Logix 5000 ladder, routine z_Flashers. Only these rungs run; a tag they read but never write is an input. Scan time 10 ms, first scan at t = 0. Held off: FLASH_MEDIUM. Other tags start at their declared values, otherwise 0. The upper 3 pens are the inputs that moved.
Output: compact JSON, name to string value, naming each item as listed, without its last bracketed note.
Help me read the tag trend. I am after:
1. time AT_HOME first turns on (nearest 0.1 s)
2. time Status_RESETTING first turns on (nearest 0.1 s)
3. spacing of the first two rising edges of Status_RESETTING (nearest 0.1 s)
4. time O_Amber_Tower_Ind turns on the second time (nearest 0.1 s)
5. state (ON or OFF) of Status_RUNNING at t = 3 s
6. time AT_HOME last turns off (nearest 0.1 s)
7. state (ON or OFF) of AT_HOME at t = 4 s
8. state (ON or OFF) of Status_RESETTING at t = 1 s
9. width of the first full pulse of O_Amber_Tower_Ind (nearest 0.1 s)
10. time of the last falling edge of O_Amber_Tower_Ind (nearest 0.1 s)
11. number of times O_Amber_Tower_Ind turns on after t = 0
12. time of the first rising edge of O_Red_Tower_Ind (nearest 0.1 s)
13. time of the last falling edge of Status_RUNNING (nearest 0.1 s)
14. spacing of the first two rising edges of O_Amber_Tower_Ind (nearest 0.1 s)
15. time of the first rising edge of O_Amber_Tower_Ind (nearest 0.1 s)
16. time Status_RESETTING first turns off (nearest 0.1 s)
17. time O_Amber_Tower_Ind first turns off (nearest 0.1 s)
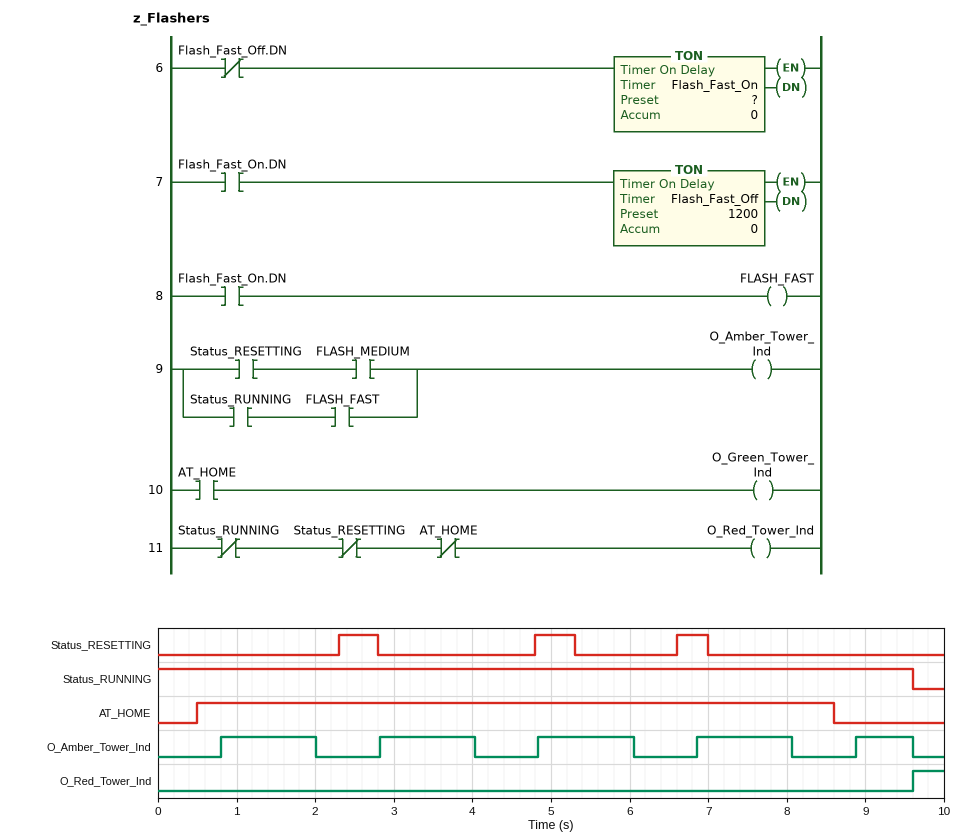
{"time AT_HOME first turns on": "0.5 s", "time Status_RESETTING first turns on": "2.3 s", "spacing of the first two rising edges of Status_RESETTING": "2.5 s", "time O_Amber_Tower_Ind turns on the second time": "2.8 s", "state (ON or OFF) of Status_RUNNING at t = 3 s": "ON", "time AT_HOME last turns off": "8.6 s", "state (ON or OFF) of AT_HOME at t = 4 s": "ON", "state (ON or OFF) of Status_RESETTING at t = 1 s": "OFF", "width of the first full pulse of O_Amber_Tower_Ind": "1.2 s", "time of the last falling edge of O_Amber_Tower_Ind": "9.6 s", "number of times O_Amber_Tower_Ind turns on after t = 0": "5", "time of the first rising edge of O_Red_Tower_Ind": "9.6 s", "time of the last falling edge of Status_RUNNING": "9.6 s", "spacing of the first two rising edges of O_Amber_Tower_Ind": "2.0 s", "time of the first rising edge of O_Amber_Tower_Ind": "0.8 s", "time Status_RESETTING first turns off": "2.8 s", "time O_Amber_Tower_Ind first turns off": "2.0 s"}
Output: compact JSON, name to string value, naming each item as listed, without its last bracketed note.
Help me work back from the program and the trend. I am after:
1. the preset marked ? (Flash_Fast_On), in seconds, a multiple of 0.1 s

{"the preset marked ? (Flash_Fast_On), in seconds, a multiple of 0.1 s": "0.8 s"}
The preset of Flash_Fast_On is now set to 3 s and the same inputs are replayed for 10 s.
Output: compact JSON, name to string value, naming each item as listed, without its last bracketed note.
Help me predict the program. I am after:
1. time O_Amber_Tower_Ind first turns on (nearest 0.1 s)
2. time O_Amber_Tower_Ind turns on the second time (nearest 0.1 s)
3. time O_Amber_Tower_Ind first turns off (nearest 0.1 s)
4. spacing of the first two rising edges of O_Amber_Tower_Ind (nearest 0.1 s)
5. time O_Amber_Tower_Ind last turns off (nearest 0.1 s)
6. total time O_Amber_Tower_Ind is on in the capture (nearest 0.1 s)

{"time O_Amber_Tower_Ind first turns on": "3.0 s", "time O_Amber_Tower_Ind turns on the second time": "7.2 s", "time O_Amber_Tower_Ind first turns off": "4.2 s", "spacing of the first two rising edges of O_Amber_Tower_Ind": "4.2 s", "time O_Amber_Tower_Ind last turns off": "8.4 s", "total time O_Amber_Tower_Ind is on in the capture": "2.4 s"}
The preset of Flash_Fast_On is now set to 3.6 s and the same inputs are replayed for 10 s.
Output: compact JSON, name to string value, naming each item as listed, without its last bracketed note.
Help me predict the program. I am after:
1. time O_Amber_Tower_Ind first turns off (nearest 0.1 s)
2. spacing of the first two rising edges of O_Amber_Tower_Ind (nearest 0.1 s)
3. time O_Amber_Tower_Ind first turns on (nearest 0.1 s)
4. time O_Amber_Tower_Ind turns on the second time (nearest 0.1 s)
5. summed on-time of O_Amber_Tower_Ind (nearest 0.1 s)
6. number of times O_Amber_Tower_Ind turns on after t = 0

{"time O_Amber_Tower_Ind first turns off": "4.8 s", "spacing of the first two rising edges of O_Amber_Tower_Ind": "4.8 s", "time O_Amber_Tower_Ind first turns on": "3.6 s", "time O_Amber_Tower_Ind turns on the second time": "8.4 s", "summed on-time of O_Amber_Tower_Ind": "2.4 s", "number of times O_Amber_Tower_Ind turns on after t = 0": "2"}
